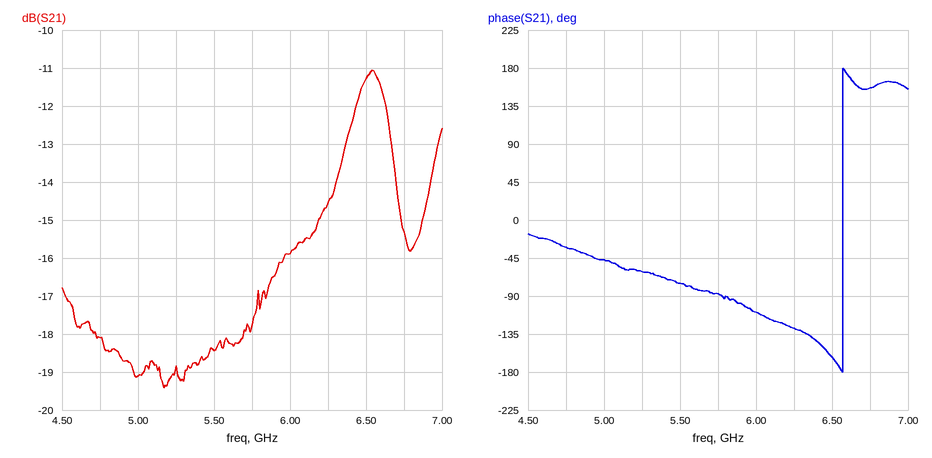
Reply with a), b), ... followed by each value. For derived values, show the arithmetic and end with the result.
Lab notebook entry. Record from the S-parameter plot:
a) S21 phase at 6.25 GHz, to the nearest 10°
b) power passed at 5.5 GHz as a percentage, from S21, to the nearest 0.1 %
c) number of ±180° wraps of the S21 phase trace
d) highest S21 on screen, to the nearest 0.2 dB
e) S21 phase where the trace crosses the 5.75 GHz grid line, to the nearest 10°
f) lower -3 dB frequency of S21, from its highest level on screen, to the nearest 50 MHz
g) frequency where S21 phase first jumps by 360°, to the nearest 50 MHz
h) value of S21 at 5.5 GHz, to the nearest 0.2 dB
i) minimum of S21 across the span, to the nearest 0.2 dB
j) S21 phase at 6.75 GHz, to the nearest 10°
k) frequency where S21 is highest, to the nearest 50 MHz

a) -130°
b) 10^(-18.4/10) ≈ 1.4 %
c) 1
d) -11.0 dB
e) -90°
f) 6.30 GHz
g) 6.55 GHz
h) -18.4 dB
i) -19.4 dB
j) 160°
k) 6.55 GHz
